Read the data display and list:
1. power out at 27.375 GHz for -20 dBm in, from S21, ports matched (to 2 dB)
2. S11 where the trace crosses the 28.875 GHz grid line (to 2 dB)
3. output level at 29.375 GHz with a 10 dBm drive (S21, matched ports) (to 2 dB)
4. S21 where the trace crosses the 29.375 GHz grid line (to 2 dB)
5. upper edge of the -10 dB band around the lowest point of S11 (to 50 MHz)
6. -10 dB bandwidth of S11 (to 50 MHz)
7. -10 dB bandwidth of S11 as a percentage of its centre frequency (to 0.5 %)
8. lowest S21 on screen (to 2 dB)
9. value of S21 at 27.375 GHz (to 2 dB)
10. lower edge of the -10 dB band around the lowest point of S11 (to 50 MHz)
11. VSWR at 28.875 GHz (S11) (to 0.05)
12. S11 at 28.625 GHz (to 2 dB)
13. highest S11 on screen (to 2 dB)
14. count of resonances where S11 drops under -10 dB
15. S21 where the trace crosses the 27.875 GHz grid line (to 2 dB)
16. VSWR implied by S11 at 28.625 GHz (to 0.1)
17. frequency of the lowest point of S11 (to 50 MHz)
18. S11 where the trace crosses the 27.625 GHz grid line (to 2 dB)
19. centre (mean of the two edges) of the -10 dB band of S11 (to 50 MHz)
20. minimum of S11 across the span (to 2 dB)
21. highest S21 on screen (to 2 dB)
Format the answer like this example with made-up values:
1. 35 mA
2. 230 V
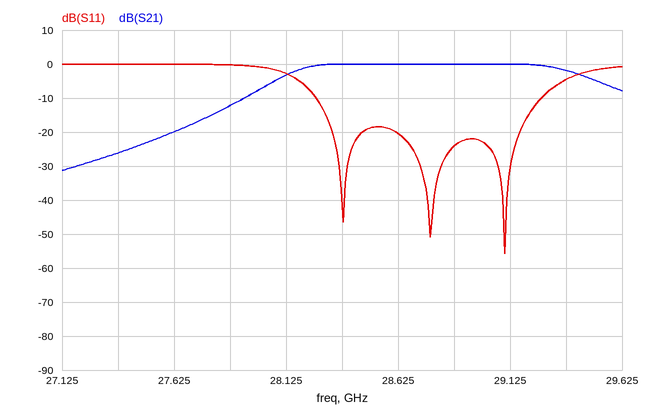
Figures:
1. -46 dBm
2. -24 dB
3. 8 dBm
4. -2 dB
5. 29.25 GHz
6. 1.00 GHz
7. 3.5 %
8. -32 dB
9. -26 dB
10. 28.25 GHz
11. 1.15
12. -20 dB
13. 0 dB
14. 3
15. -12 dB
16. 1.2
17. 29.10 GHz
18. 0 dB
19. 28.75 GHz
20. -56 dB
21. 0 dB
